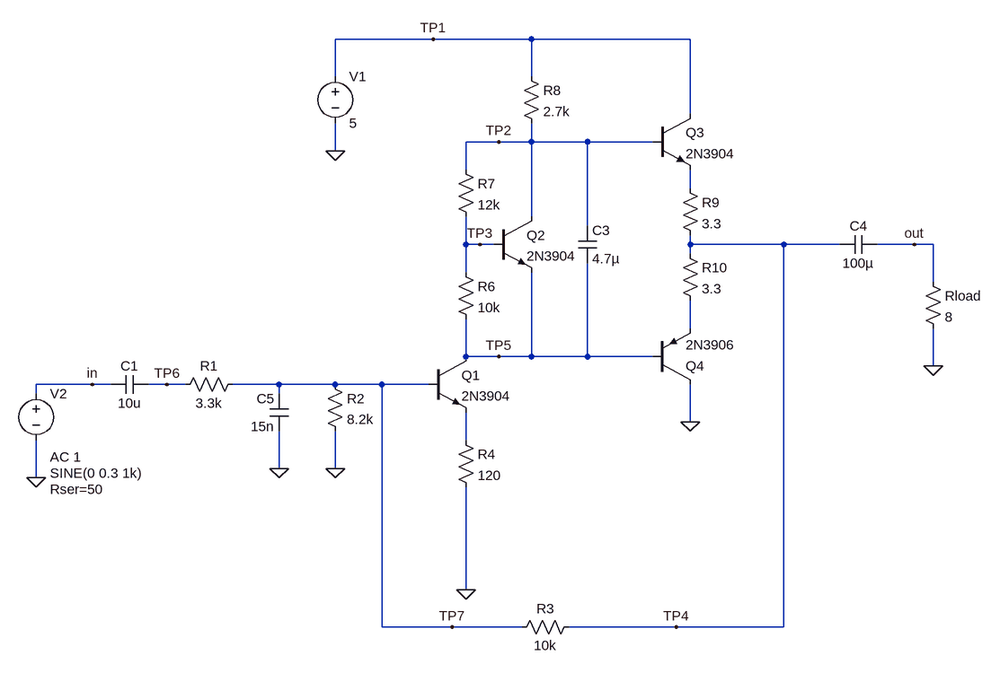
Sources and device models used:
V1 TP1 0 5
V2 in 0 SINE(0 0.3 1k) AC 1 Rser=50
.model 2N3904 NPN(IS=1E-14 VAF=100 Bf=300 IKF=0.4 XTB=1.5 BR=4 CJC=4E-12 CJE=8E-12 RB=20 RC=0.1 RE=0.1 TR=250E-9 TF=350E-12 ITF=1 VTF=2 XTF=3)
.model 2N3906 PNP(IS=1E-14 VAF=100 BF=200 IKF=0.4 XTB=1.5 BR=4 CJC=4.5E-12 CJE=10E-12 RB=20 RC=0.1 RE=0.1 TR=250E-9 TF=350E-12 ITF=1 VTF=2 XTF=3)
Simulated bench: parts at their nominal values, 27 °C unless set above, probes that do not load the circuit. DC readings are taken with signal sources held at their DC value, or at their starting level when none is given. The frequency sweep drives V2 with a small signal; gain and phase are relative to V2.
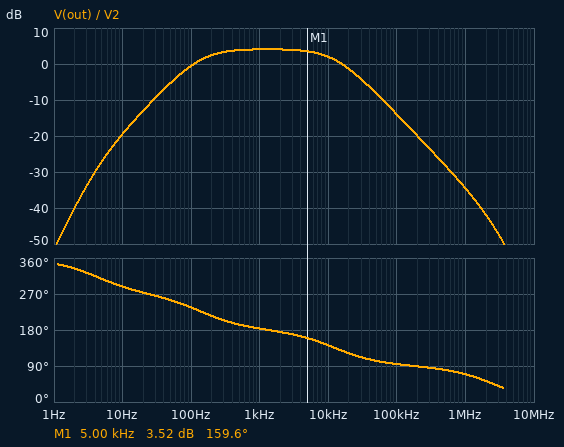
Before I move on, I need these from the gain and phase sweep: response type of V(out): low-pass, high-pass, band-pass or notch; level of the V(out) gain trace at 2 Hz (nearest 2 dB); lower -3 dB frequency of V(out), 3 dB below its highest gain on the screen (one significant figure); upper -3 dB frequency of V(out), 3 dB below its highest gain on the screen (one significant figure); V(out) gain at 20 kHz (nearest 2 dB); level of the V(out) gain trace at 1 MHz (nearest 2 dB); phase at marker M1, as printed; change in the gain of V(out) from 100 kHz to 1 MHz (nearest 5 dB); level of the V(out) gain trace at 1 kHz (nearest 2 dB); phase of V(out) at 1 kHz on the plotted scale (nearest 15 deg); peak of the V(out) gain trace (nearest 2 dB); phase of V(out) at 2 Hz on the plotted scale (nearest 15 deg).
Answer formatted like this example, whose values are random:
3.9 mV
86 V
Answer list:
band-pass
-40 dB
100 Hz
10 kHz
-2 dB
-34 dB
159.6 deg
-20 dB
4 dB
180 deg
4 dB
330 deg
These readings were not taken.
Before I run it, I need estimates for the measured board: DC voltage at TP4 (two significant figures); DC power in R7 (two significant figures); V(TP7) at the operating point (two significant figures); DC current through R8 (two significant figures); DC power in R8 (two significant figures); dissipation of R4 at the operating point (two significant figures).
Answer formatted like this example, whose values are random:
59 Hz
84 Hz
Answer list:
1.7 V
55 µW
770 mV
940 µA
2.4 mW
110 µW
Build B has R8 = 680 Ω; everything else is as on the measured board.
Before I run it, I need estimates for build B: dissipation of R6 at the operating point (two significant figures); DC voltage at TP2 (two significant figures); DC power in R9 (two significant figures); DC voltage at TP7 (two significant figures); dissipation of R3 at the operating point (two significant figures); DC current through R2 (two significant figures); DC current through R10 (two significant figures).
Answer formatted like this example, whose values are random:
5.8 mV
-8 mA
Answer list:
46 µW
3.1 V
1.2 mW
1.0 V
180 µW
120 µA
19 mA
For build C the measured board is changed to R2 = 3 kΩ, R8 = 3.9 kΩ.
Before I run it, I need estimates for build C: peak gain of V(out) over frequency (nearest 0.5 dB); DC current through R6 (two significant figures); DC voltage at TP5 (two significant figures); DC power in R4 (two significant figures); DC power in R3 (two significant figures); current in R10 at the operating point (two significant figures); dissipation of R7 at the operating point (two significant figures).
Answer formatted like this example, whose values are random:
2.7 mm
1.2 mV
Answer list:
2.0 dB
62 µA
2.2 V
16 µW
510 µW
2.6 mA
48 µW
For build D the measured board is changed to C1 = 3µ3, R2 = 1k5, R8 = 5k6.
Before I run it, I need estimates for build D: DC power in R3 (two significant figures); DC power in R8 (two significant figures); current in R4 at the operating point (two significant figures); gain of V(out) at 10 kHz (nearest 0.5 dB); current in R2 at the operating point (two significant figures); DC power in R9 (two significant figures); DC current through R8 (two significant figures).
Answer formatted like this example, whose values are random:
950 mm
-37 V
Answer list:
1.4 mW
2.4 µW
20 µA
-24.0 dB
370 µA
450 nW
21 µA
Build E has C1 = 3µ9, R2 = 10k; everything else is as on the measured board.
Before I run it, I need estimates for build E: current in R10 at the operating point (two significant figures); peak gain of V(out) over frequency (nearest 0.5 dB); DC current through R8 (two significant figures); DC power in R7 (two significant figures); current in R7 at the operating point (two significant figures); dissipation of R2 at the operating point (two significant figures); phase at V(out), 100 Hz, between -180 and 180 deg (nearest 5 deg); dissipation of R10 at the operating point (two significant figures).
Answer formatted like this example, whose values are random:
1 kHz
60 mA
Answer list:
7.8 mA
4.5 dB
990 µA
56 µW
68 µA
60 µW
-120 deg
200 µW
